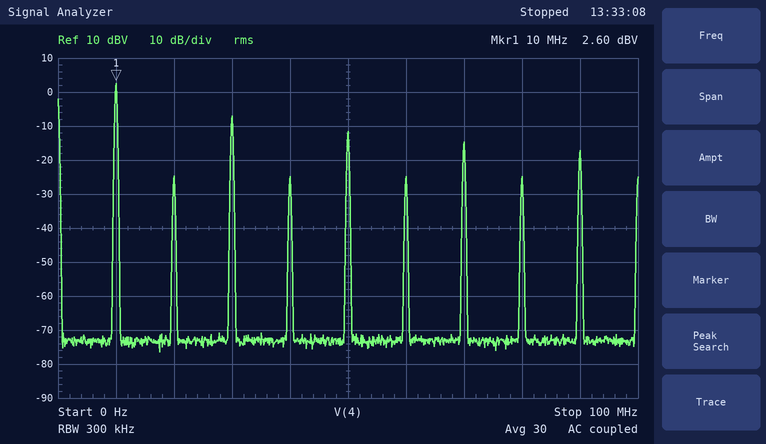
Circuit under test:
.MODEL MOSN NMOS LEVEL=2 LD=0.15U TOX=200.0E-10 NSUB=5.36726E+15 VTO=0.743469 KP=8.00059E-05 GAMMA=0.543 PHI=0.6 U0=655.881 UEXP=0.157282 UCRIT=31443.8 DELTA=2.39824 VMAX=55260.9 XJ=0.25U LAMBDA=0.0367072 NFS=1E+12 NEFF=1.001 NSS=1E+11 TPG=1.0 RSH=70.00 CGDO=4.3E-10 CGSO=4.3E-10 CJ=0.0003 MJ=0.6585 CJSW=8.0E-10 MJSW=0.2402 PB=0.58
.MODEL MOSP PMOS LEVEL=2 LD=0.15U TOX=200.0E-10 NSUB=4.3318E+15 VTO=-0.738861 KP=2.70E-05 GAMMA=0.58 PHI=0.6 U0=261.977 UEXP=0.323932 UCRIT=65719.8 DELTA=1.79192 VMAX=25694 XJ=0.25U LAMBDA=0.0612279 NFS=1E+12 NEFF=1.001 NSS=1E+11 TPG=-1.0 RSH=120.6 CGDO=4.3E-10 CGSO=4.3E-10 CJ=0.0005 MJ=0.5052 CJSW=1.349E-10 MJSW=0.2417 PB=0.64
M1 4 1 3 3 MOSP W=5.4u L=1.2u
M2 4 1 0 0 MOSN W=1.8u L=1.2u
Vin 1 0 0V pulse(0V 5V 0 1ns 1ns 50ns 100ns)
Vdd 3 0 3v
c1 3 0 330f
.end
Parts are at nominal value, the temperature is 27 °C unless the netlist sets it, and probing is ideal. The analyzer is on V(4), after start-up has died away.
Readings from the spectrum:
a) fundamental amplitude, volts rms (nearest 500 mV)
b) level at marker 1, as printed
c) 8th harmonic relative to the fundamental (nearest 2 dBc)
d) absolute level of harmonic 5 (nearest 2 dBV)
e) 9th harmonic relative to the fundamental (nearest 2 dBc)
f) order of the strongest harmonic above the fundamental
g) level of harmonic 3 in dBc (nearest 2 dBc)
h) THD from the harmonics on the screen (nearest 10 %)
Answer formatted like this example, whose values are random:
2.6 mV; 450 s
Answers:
1.5 V; 2.60 dBV; -28 dBc; -12 dBV; -20 dBc; 3; -10 dBc; 40 %
